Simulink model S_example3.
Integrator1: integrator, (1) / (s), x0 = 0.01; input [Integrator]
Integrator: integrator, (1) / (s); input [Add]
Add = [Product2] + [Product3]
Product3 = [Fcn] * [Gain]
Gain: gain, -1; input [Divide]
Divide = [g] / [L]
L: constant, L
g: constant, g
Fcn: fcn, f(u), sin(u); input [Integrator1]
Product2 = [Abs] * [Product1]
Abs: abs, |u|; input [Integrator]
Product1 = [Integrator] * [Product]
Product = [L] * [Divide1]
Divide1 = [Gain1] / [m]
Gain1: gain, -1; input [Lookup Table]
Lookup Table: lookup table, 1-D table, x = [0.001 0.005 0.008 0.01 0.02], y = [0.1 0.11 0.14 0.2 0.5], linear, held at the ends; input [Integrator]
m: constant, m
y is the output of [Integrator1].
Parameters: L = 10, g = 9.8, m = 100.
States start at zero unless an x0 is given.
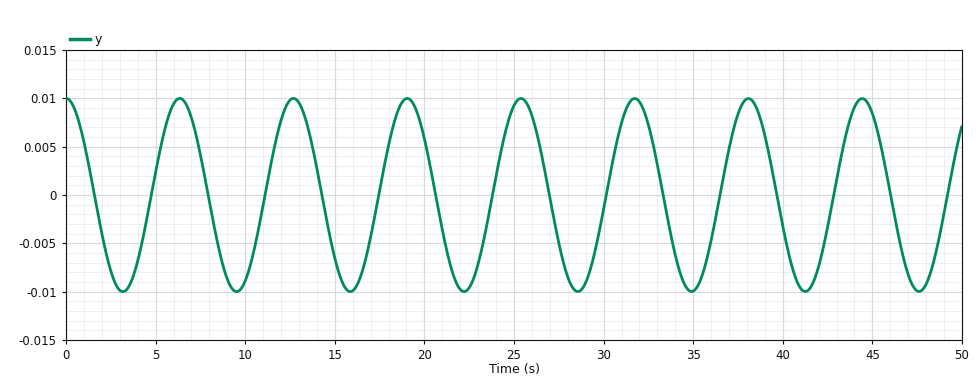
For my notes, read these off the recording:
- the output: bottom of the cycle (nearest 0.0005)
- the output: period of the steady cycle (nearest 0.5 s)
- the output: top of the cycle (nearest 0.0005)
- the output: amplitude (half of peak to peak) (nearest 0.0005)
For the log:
-0.0100
6.5 s
0.0100
0.0100
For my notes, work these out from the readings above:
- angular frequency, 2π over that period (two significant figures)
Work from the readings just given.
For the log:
0.97 rad/s
